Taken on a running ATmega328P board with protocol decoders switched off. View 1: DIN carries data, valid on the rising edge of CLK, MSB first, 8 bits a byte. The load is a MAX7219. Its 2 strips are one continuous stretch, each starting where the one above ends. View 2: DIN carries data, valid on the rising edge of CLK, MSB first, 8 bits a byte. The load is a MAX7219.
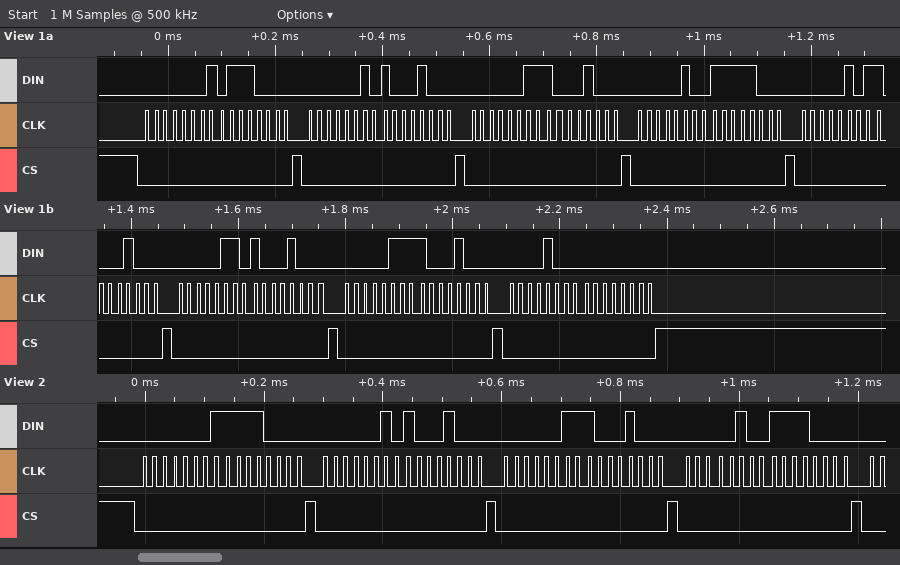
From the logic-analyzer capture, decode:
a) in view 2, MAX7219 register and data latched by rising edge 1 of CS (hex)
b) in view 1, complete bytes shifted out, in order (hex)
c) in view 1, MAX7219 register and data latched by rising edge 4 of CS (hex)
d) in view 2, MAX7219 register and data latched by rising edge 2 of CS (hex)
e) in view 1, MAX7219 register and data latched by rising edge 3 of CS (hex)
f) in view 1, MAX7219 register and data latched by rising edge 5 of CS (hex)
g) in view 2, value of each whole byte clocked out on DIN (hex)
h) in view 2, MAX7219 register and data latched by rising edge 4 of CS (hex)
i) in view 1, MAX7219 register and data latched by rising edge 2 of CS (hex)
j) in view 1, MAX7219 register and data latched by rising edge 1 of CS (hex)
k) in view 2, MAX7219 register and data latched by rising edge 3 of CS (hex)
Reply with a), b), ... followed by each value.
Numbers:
a) register 0x1, data 0xF0
b) 01 70 02 88 03 88 04 F8 05 88 06 88 07 88 08 00
c) register 0x4, data 0xF8
d) register 0x2, data 0x88
e) register 0x3, data 0x88
f) register 0x5, data 0x88
g) 0x01 0xF0 0x02 0x88 0x03 0x88 0x04 0xF0
h) register 0x4, data 0xF0
i) register 0x2, data 0x88
j) register 0x1, data 0x70
k) register 0x3, data 0x88
